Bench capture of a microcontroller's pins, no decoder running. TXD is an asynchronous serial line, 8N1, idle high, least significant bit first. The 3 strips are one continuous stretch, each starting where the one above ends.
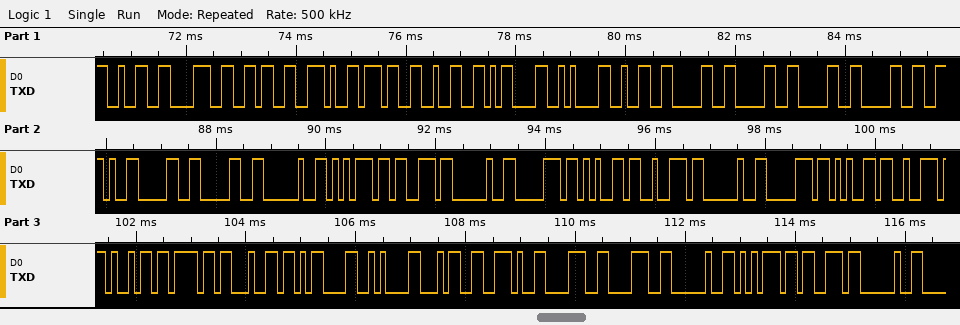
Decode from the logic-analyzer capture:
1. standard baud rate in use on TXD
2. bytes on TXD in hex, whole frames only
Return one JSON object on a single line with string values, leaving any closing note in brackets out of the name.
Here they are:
{"standard baud rate in use on TXD": "9600 baud", "bytes on TXD in hex, whole frames only": "32 38 36 2E 37 32 0D 0A 32 30 30 30 30 2E 30 30 20 75 73 20 70 65 72 20 70 65 72 69 6F 64 0D 0A 34 2E 38 38 20 75 73 20"}
